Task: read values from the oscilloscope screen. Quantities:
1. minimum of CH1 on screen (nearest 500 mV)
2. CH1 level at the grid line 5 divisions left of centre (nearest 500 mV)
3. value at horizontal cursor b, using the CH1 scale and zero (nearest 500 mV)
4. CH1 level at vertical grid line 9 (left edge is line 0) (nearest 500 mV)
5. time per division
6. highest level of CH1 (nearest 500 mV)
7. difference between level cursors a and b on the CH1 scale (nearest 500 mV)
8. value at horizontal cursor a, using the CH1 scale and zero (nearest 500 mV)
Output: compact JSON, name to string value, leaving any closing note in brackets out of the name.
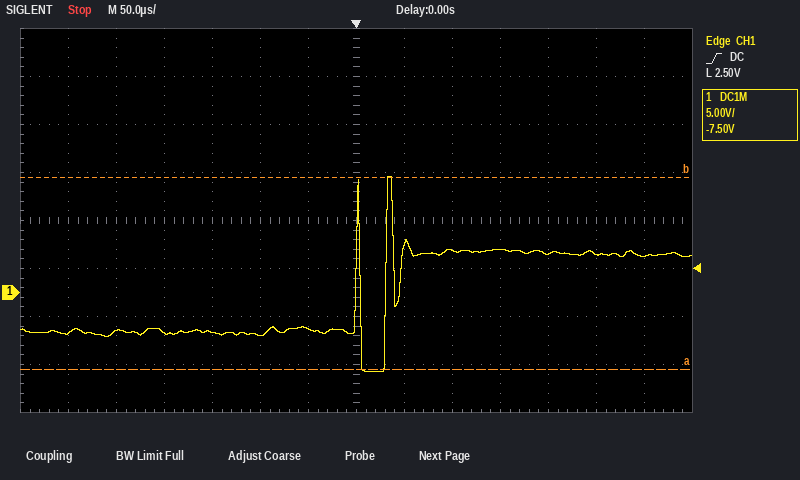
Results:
{"minimum of CH1 on screen": "-8.0 V", "CH1 level at the grid line 5 divisions left of centre": "-4.0 V", "value at horizontal cursor b, using the CH1 scale and zero": "12.0 V", "CH1 level at vertical grid line 9 (left edge is line 0)": "4.5 V", "time per division": "50 µs", "highest level of CH1": "12.0 V", "difference between level cursors a and b on the CH1 scale": "20.0 V", "value at horizontal cursor a, using the CH1 scale and zero": "-8.0 V"}
